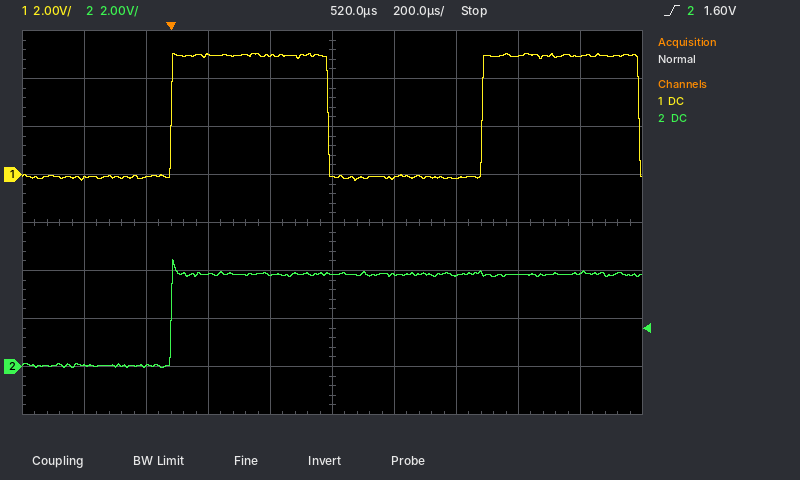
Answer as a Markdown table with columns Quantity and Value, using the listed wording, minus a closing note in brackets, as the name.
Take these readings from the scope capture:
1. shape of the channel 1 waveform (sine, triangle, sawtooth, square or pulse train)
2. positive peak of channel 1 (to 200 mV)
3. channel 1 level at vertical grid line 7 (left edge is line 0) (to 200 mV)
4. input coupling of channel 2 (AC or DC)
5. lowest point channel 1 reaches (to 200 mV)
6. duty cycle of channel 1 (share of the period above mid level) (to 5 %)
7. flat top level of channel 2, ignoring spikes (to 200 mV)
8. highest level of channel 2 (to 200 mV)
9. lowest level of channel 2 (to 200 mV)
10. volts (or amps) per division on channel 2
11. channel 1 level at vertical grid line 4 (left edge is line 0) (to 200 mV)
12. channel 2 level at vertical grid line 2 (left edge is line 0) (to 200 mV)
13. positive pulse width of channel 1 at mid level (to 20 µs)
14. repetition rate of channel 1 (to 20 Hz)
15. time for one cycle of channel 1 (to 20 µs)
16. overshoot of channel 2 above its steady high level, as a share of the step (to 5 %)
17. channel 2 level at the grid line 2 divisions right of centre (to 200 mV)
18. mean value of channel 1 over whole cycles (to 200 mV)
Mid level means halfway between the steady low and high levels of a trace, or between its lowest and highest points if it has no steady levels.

| Quantity | Value |
|---|---|
| shape of the channel 1 waveform | square |
| positive peak of channel 1 | 5.0 V |
| channel 1 level at vertical grid line 7 (left edge is line 0) | -200 mV |
| input coupling of channel 2 | DC |
| lowest point channel 1 reaches | -200 mV |
| duty cycle of channel 1 (share of the period above mid level) | 50 % |
| flat top level of channel 2, ignoring spikes | 3.8 V |
| highest level of channel 2 | 4.4 V |
| lowest level of channel 2 | 0.0 V |
| volts (or amps) per division on channel 2 | 2 V |
| channel 1 level at vertical grid line 4 (left edge is line 0) | 5.0 V |
| channel 2 level at vertical grid line 2 (left edge is line 0) | 0.0 V |
| positive pulse width of channel 1 at mid level | 500 µs |
| repetition rate of channel 1 | 1.00 kHz |
| time for one cycle of channel 1 | 1.00 ms |
| overshoot of channel 2 above its steady high level, as a share of the step | 15 % |
| channel 2 level at the grid line 2 divisions right of centre | 3.8 V |
| mean value of channel 1 over whole cycles | 2.4 V |
